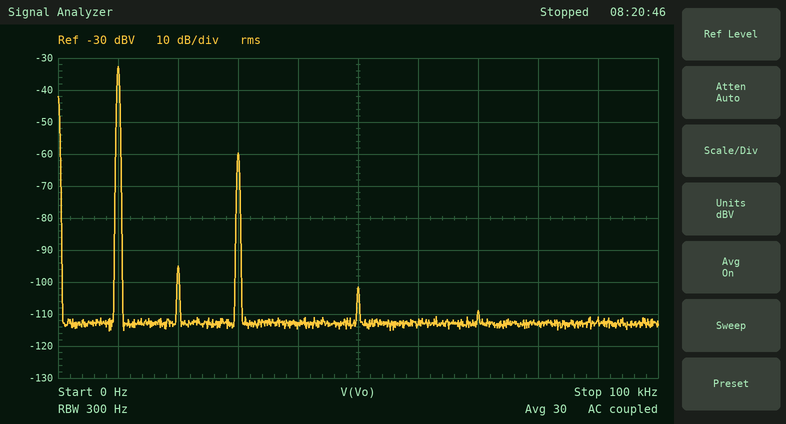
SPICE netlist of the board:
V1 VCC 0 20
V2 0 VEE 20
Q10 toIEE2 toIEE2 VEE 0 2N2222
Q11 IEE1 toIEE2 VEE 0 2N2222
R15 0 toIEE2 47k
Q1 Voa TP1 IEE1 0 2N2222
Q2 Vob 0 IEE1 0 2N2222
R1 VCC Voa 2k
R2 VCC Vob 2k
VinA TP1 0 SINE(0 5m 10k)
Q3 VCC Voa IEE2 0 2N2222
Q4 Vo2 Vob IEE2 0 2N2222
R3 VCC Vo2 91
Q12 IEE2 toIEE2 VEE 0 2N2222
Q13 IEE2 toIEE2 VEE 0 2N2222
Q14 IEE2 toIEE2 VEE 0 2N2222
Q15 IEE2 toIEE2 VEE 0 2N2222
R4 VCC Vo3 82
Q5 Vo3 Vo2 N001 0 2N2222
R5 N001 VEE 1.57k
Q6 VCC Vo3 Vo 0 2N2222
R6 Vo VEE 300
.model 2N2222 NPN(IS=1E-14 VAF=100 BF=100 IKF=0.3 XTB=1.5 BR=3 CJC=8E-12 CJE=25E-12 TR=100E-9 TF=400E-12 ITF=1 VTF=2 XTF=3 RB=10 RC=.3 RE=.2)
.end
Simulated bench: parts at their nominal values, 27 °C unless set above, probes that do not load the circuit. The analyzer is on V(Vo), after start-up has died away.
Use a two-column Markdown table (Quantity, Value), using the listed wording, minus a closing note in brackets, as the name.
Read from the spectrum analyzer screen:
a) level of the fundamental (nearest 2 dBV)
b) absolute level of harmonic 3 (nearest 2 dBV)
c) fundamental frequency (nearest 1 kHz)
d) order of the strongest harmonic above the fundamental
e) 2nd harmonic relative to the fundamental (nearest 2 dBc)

| Quantity | Value |
|---|---|
| level of the fundamental | -32 dBV |
| absolute level of harmonic 3 | -60 dBV |
| fundamental frequency | 10 kHz |
| order of the strongest harmonic above the fundamental | 3 |
| 2nd harmonic relative to the fundamental | -62 dBc |
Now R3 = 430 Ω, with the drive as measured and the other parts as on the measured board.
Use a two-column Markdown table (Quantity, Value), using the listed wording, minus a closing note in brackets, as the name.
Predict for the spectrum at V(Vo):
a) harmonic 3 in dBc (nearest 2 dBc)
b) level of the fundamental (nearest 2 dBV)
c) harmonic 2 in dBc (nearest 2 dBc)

| Quantity | Value |
|---|---|
| harmonic 3 in dBc | -38 dBc |
| level of the fundamental | -44 dBV |
| harmonic 2 in dBc | -12 dBc |
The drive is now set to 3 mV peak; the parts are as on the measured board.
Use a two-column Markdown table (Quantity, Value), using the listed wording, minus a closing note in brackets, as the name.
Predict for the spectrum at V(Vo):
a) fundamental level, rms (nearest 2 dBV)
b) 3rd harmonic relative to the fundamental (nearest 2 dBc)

| Quantity | Value |
|---|---|
| fundamental level, rms | -36 dBV |
| 3rd harmonic relative to the fundamental | -36 dBc |
